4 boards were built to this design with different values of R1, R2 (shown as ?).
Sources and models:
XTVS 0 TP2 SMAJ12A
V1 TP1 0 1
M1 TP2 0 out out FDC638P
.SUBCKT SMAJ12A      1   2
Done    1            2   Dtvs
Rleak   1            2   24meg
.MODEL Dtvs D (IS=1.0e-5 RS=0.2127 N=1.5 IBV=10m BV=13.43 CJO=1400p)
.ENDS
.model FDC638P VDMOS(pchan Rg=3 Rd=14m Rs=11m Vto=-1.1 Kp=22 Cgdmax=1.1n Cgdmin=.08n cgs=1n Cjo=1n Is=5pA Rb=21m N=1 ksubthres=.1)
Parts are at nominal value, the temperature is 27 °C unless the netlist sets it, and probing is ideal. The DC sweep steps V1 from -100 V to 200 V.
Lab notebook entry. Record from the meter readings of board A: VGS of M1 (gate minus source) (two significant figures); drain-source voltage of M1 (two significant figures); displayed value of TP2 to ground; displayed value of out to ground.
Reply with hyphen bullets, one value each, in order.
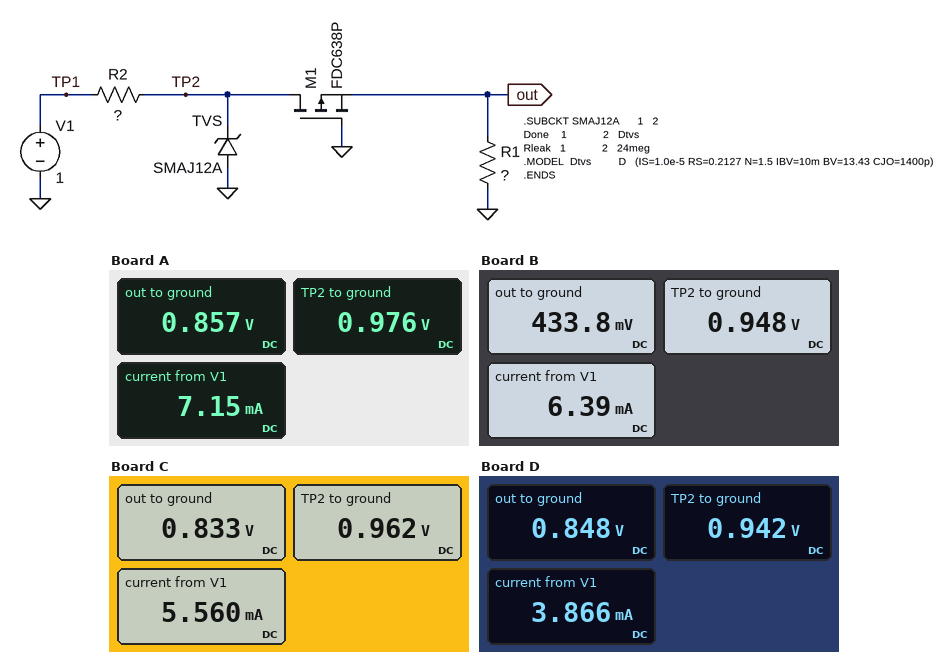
- -860 mV
- 120 mV
- 0.976 V
- 0.857 V
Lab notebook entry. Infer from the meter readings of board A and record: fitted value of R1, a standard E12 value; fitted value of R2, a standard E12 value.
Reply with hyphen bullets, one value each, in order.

- 120 Ω
- 3.3 Ω
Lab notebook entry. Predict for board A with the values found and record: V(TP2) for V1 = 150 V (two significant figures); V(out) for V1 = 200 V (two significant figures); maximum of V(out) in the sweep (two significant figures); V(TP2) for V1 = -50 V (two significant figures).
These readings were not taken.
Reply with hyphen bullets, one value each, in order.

- 22 V
- 25 V
- 25 V
- -3.5 V
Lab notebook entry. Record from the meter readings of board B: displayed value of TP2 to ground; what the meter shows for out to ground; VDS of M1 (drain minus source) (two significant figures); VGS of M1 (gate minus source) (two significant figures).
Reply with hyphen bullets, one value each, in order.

- 0.948 V
- 433.8 mV
- 510 mV
- -430 mV
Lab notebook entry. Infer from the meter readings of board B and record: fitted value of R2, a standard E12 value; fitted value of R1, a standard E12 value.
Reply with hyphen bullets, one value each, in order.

- 8.2 Ω
- 68 Ω
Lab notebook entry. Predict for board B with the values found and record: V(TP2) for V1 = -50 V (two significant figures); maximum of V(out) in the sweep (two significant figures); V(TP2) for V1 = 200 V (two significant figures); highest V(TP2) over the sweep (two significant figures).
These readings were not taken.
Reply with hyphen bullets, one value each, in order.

- -1.8 V
- 18 V
- 18 V
- 18 V
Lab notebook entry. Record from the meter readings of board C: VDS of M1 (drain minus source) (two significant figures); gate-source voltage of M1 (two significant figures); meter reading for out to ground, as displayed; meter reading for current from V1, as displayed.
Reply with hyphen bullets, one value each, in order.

- 130 mV
- -830 mV
- 0.833 V
- 5.560 mA
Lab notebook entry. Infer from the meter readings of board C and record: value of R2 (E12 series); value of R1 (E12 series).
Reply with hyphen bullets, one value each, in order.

- 6.8 Ω
- 150 Ω
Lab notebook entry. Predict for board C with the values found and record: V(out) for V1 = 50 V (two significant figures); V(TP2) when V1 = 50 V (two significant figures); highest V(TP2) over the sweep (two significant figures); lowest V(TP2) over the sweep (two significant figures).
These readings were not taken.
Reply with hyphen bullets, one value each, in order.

- 15 V
- 15 V
- 19 V
- -3.6 V
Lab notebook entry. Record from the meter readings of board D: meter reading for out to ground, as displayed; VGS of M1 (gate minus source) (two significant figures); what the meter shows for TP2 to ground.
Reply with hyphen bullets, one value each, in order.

- 0.848 V
- -850 mV
- 0.942 V
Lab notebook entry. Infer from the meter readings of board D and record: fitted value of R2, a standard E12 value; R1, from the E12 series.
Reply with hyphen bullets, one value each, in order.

- 15 Ω
- 220 Ω
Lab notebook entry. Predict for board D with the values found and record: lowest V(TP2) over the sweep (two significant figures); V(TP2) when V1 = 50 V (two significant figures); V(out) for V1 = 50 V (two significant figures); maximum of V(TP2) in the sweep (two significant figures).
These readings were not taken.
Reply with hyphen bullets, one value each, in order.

- -1.9 V
- 14 V
- 14 V
- 16 V
